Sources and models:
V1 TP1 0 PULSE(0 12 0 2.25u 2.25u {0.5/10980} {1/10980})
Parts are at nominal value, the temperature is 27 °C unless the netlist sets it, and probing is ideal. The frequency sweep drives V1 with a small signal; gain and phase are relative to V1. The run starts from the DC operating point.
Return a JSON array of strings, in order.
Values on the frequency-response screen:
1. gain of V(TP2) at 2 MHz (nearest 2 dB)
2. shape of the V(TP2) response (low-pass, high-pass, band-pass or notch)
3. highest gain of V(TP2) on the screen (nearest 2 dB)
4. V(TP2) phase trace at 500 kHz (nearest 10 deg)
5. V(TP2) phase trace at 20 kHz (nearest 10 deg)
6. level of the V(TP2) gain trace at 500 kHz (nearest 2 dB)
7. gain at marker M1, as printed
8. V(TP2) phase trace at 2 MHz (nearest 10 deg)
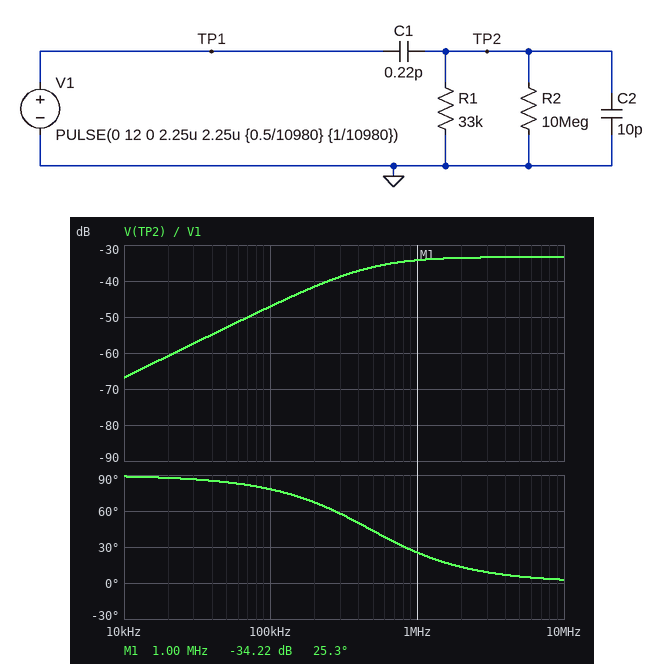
["-34 dB", "high-pass", "-34 dB", "40 deg", "90 deg", "-36 dB", "-34.22 dB", "10 deg"]
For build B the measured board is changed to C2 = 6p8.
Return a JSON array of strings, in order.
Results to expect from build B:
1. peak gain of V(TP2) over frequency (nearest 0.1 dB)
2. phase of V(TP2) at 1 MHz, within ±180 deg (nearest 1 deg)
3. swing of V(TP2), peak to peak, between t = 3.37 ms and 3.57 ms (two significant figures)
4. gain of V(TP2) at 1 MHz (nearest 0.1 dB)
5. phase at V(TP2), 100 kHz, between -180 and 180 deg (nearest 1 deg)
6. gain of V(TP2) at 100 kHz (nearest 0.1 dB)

["-30.1 dB", "35 deg", "77 mV", "-31.8 dB", "82 deg", "-46.9 dB"]
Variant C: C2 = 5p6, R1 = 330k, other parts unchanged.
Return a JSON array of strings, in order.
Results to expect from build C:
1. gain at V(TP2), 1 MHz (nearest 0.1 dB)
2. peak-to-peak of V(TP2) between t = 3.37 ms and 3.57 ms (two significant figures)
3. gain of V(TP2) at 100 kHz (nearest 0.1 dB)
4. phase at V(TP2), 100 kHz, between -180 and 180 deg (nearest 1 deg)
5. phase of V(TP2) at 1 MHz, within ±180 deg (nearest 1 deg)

["-28.5 dB", "530 mV", "-30.8 dB", "41 deg", "5 deg"]
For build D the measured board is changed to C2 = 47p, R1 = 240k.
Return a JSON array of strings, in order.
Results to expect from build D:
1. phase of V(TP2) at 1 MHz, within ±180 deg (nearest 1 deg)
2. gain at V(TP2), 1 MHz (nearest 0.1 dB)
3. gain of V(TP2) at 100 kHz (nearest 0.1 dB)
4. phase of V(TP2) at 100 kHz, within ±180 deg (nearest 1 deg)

["1 deg", "-46.6 dB", "-46.7 dB", "8 deg"]
